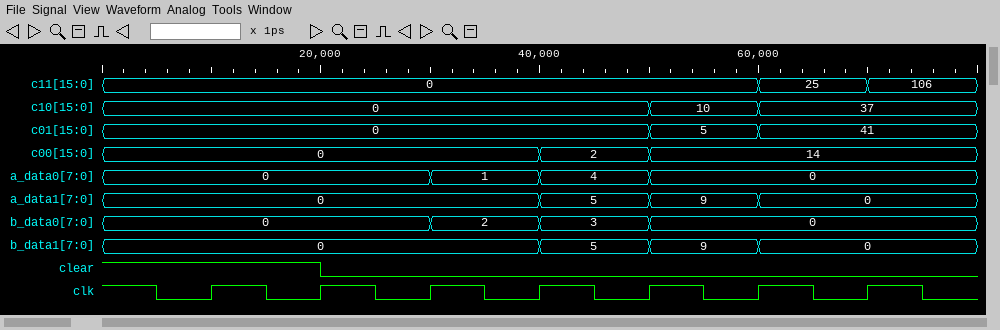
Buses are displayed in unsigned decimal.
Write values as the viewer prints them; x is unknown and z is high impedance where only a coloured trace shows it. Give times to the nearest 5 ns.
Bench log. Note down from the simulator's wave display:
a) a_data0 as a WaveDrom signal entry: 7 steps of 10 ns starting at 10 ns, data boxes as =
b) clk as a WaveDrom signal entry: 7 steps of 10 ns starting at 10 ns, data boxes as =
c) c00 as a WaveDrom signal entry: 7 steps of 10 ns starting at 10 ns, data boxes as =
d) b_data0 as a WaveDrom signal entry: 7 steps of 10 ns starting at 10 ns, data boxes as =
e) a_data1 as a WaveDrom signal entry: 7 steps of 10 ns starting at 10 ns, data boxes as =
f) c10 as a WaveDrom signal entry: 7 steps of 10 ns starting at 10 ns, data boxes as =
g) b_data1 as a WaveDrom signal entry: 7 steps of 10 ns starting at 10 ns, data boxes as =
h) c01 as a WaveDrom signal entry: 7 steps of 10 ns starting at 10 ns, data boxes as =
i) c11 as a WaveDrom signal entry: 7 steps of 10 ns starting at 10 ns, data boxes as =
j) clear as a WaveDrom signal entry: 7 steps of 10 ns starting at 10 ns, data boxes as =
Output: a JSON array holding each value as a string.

["{name: 'a_data0', wave: '=.===..', data: '0 1 4 0'}", "{name: 'clk', wave: 'p......'}", "{name: 'c00', wave: '=..==..', data: '0 2 14'}", "{name: 'b_data0', wave: '=.===..', data: '0 2 3 0'}", "{name: 'a_data1', wave: '=..===.', data: '0 5 9 0'}", "{name: 'c10', wave: '=...==.', data: '0 10 37'}", "{name: 'b_data1', wave: '=..===.', data: '0 5 9 0'}", "{name: 'c01', wave: '=...==.', data: '0 5 41'}", "{name: 'c11', wave: '=....==', data: '0 25 106'}", "{name: 'clear', wave: '10.....'}"]
